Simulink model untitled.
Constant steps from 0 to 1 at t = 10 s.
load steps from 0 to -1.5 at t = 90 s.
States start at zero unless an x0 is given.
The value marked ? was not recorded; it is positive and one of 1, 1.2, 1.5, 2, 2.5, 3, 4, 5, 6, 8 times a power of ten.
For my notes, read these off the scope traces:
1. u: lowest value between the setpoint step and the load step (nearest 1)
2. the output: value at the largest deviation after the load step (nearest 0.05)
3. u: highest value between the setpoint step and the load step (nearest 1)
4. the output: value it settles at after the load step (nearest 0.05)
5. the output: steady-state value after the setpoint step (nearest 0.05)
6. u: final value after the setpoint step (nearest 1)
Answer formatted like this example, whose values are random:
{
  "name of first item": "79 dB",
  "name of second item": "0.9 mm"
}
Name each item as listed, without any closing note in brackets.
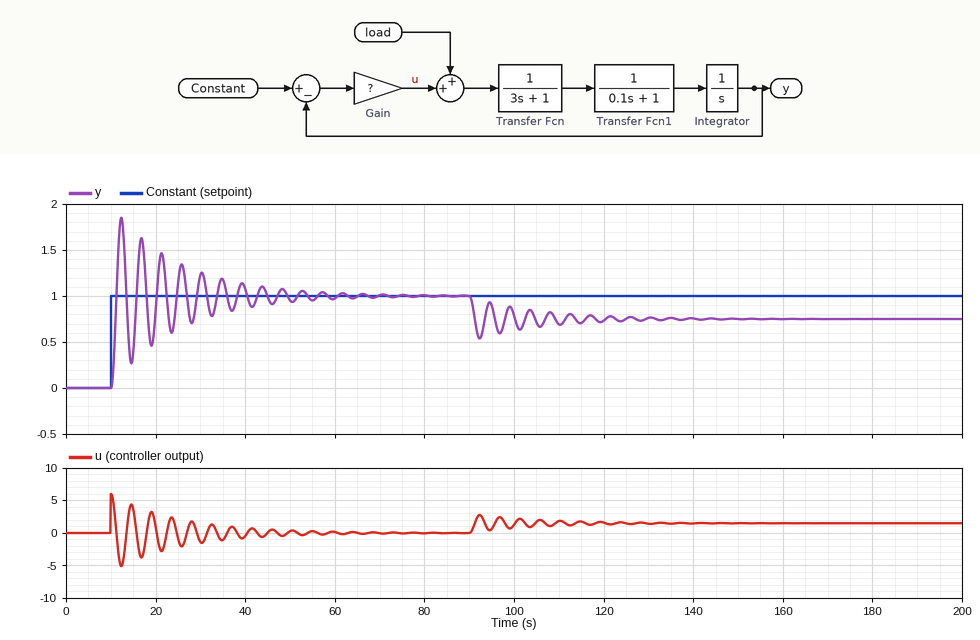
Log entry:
{
  "u: lowest value between the setpoint step and the load step": "-5",
  "the output: value at the largest deviation after the load step": "0.55",
  "u: highest value between the setpoint step and the load step": "6",
  "the output: value it settles at after the load step": "0.75",
  "the output: steady-state value after the setpoint step": "1.00",
  "u: final value after the setpoint step": "0"
}
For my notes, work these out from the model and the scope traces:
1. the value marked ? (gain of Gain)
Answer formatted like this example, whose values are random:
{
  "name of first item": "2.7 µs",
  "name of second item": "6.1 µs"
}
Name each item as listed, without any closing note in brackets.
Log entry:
{
  "the value marked ?": "6"
}
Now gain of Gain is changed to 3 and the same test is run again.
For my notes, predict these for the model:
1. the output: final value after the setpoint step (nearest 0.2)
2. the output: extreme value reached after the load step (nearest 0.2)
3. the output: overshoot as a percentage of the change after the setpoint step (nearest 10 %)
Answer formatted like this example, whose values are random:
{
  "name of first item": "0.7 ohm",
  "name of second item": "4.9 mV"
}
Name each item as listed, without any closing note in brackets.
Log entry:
{
  "the output: final value after the setpoint step": "1.0",
  "the output: extreme value reached after the load step": "0.2",
  "the output: overshoot as a percentage of the change after the setpoint step": "70 %"
}
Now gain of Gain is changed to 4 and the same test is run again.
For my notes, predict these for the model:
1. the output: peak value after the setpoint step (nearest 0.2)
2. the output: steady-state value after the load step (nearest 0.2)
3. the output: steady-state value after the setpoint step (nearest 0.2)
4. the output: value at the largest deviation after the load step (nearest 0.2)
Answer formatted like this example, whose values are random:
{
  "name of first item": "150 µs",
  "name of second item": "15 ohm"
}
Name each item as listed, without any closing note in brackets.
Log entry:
{
  "the output: peak value after the setpoint step": "1.8",
  "the output: steady-state value after the load step": "0.6",
  "the output: steady-state value after the setpoint step": "1.0",
  "the output: value at the largest deviation after the load step": "0.4"
}
